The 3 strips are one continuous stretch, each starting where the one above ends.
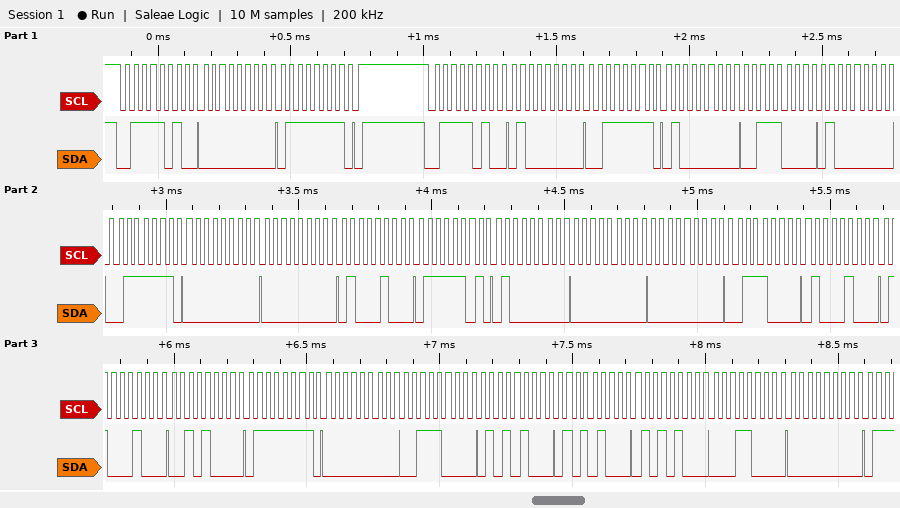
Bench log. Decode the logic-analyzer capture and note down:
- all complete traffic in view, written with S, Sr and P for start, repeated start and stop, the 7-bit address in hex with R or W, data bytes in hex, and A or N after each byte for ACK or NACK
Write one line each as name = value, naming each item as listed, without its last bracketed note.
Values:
all complete traffic in view, written with S, Sr and P for start, repeated start and stop, the 7-bit address in hex with R or W, data bytes in hex, and A or N after each byte for ACK or NACK = S 3DW A 00 A 7F A P S 3DW A 40 A 3F A 40 A 38 A 40 A 3F A 00 A 00 A 44 A 7D A 40 A 00 A 00 A 38 A 44 A 44 A 28 A 7F A 00 A 38 A 54 A 54 A 54 A 18 A 00 A
